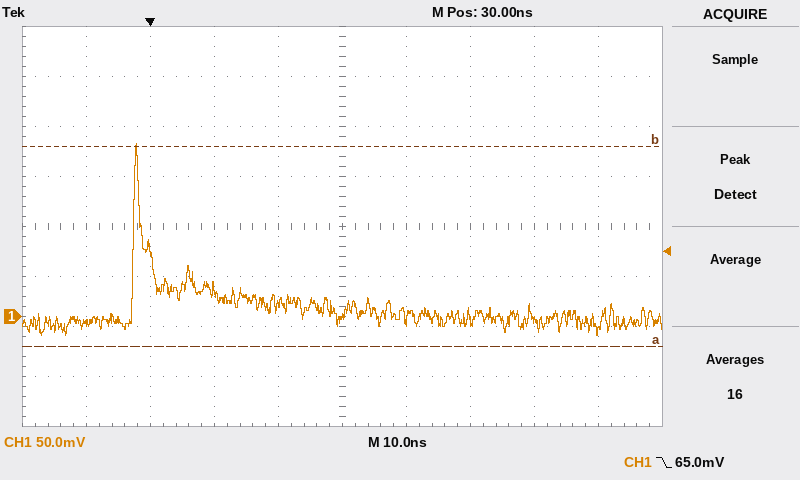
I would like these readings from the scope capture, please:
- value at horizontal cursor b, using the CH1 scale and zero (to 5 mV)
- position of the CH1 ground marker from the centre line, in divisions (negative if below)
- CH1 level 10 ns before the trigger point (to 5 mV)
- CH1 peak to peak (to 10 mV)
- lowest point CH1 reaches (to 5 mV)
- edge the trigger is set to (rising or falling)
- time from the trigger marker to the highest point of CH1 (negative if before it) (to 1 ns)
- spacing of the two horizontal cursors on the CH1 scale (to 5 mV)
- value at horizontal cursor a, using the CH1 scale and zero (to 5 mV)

170 mV
-1.8 div
-5 mV
190 mV
-20 mV
falling
-2 ns
200 mV
-30 mV
